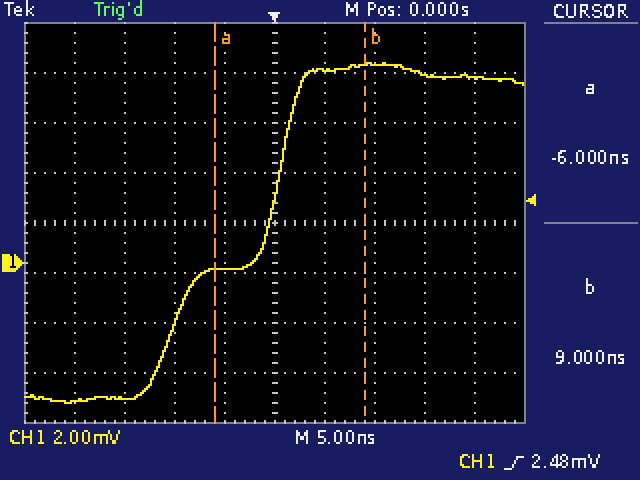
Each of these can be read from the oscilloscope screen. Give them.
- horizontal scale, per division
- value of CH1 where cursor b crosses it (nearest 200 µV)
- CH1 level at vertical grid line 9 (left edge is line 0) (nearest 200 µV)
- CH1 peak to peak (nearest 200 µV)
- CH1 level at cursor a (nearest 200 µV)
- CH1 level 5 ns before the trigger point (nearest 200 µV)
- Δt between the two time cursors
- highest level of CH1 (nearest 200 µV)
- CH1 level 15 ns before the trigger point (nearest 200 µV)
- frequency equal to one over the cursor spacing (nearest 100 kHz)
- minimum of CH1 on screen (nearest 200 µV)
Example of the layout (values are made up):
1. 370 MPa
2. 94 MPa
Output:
1. 5 ns
2. 8.0 mV
3. 7.4 mV
4. 13.6 mV
5. -200 µV
6. -200 µV
7. 15.0 ns
8. 8.0 mV
9. -5.4 mV
10. 66.7 MHz
11. -5.6 mV
